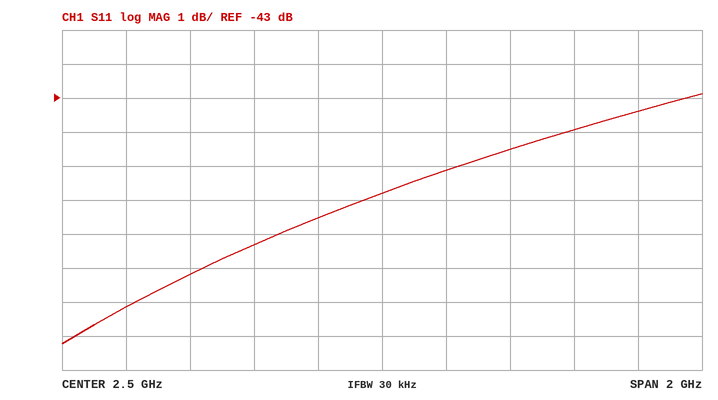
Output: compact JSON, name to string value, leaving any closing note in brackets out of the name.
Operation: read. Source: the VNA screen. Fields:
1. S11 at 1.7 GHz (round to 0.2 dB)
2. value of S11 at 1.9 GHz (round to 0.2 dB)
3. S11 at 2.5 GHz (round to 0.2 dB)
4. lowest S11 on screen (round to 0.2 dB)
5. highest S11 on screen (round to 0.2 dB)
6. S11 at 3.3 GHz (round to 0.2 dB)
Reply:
{"S11 at 1.7 GHz": "-49.2 dB", "value of S11 at 1.9 GHz": "-48.2 dB", "S11 at 2.5 GHz": "-45.8 dB", "lowest S11 on screen": "-50.2 dB", "highest S11 on screen": "-42.8 dB", "S11 at 3.3 GHz": "-43.4 dB"}
